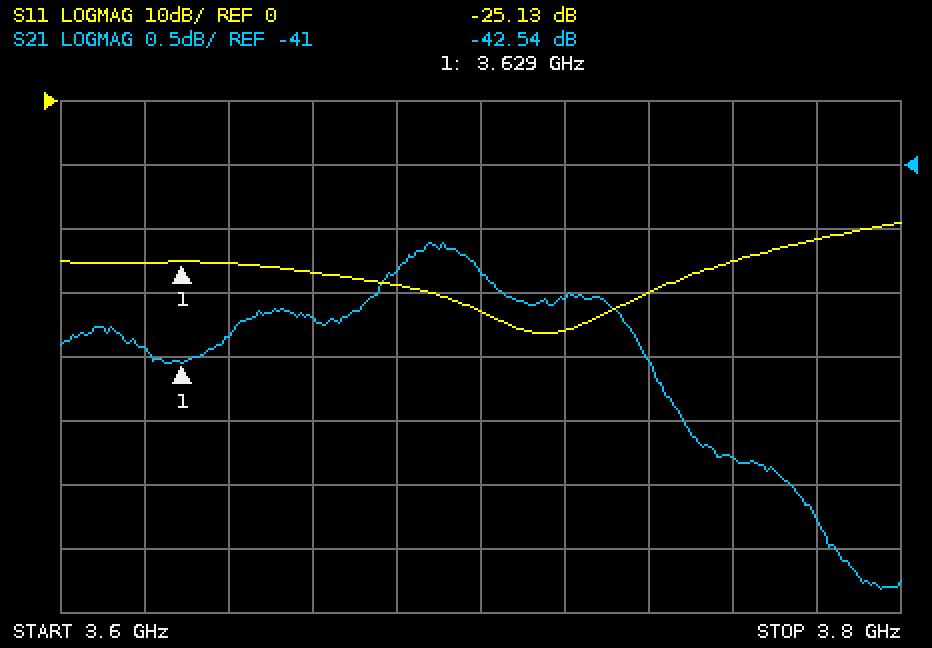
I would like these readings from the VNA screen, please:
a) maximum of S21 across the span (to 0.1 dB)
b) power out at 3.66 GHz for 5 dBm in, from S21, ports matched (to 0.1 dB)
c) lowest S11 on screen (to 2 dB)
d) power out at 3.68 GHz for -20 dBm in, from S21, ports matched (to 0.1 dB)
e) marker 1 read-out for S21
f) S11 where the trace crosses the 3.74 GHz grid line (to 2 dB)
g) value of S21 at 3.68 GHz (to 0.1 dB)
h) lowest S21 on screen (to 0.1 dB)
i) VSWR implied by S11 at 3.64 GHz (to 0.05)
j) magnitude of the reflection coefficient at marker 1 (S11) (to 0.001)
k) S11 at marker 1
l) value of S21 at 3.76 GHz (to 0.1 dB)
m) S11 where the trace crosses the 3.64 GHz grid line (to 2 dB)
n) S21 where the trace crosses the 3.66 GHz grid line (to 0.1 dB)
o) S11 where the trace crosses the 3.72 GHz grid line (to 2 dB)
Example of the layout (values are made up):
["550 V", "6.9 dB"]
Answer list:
["-41.6 dB", "-37.2 dBm", "-36 dB", "-61.8 dBm", "-42.54 dB", "-30 dB", "-41.8 dB", "-44.3 dB", "1.10", "0.055", "-25.13 dB", "-43.3 dB", "-26 dB", "-42.2 dB", "-36 dB"]
